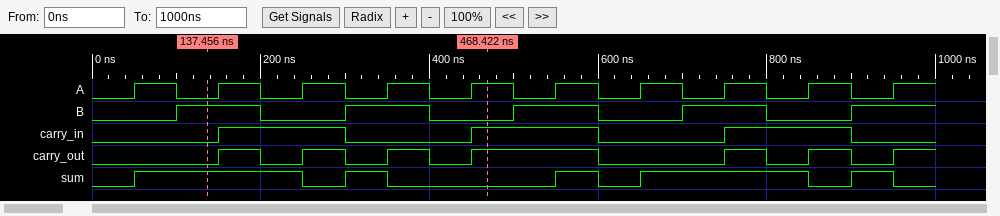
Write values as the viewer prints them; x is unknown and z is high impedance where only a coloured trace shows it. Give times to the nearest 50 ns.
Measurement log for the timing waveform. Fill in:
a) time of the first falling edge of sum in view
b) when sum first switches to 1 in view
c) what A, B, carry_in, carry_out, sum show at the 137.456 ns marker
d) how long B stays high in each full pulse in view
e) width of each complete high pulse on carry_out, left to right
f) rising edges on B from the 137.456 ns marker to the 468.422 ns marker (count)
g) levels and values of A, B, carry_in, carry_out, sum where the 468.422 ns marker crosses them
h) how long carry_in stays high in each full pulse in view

250 ns
50 ns
A=0, B=1, carry_in=0, carry_out=0, sum=1
100 ns, 100 ns, 100 ns, 100 ns
50 ns, 50 ns, 50 ns, 150 ns, 50 ns, 50 ns
1
A=1, B=0, carry_in=1, carry_out=1, sum=0
150 ns, 150 ns, 150 ns
